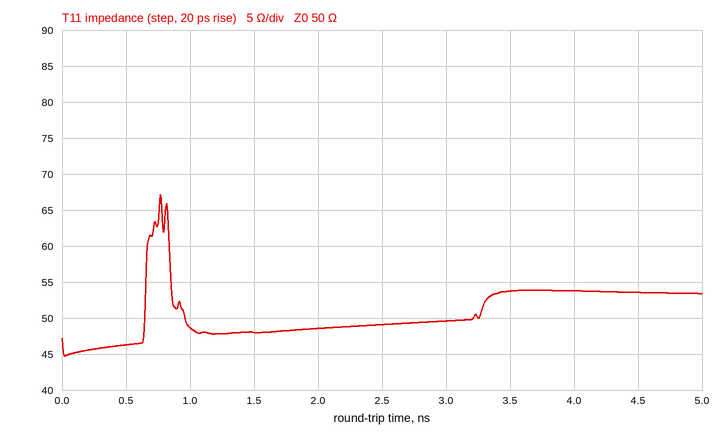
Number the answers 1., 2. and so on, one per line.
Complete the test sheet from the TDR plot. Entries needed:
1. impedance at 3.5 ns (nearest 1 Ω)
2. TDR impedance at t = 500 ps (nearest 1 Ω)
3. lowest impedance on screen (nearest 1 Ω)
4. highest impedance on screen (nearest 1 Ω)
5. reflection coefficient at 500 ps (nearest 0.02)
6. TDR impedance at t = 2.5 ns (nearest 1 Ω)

1. 54 Ω
2. 46 Ω
3. 45 Ω
4. 67 Ω
5. -0.04
6. 49 Ω
